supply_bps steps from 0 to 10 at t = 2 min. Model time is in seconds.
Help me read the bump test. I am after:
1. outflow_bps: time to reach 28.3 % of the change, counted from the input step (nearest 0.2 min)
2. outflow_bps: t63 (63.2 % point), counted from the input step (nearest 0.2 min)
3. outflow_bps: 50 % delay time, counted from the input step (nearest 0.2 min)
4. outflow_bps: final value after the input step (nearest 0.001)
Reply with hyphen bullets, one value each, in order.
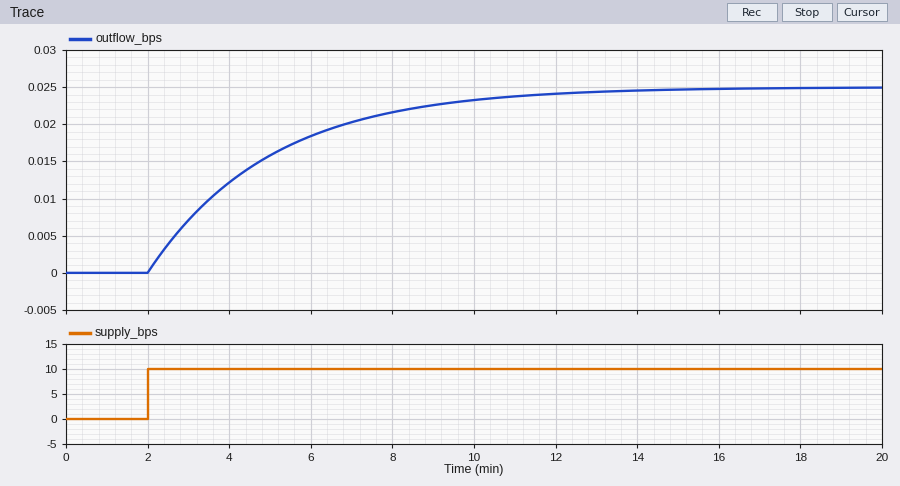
- 1.0 min
- 3.0 min
- 2.0 min
- 0.025
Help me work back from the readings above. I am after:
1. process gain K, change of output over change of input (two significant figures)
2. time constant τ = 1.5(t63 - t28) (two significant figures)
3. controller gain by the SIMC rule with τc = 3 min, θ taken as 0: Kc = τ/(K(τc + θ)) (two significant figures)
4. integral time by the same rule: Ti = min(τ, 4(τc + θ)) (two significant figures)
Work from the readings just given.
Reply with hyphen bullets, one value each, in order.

- 0.0025
- 3.0 min
- 400
- 3.0 min
